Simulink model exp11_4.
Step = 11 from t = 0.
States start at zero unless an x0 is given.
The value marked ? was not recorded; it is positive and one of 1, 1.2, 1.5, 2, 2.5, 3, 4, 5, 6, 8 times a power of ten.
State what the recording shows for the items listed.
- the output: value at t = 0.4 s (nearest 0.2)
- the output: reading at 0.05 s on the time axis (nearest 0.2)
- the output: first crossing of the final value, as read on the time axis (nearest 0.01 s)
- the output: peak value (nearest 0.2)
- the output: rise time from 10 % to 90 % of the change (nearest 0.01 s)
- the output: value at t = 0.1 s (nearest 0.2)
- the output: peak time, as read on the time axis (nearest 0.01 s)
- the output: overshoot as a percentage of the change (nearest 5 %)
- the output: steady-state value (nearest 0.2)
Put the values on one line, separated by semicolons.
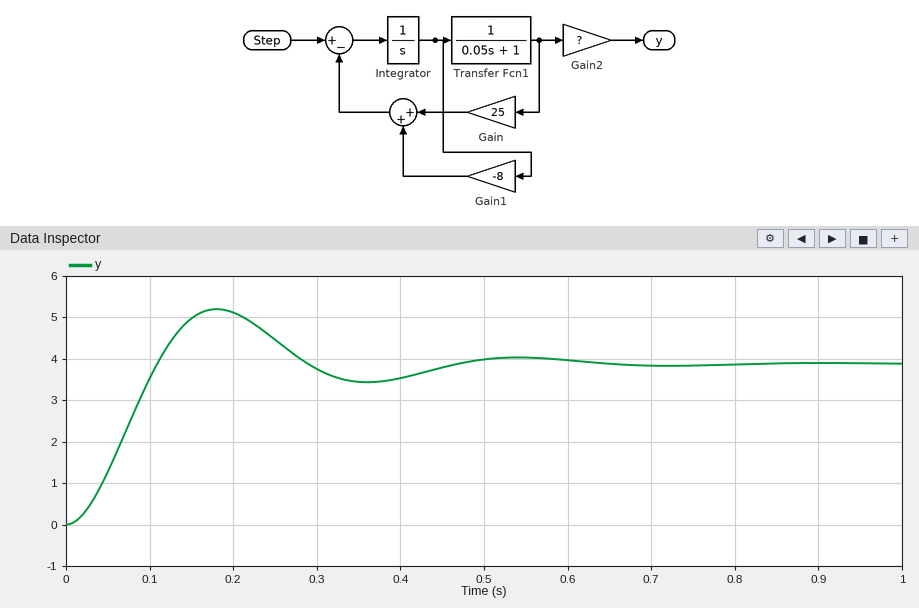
3.6; 1.2; 0.11 s; 5.2; 0.07 s; 3.6; 0.18 s; 35 %; 3.8
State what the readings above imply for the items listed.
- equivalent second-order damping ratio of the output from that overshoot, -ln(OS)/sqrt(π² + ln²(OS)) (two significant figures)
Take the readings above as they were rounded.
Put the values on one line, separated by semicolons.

0.32
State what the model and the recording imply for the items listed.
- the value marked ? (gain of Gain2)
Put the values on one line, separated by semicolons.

6
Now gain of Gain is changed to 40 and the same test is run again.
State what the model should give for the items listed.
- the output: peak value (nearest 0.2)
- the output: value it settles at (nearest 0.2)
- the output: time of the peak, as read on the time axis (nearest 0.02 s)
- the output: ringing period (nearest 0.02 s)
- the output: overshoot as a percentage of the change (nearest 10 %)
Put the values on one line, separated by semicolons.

3.0; 2.0; 0.12 s; 0.26 s; 50 %
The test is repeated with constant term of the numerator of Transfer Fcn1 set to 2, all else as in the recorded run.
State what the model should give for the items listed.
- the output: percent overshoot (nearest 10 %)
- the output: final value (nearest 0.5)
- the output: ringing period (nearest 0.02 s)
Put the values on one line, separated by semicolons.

50 %; 3.0; 0.22 s
